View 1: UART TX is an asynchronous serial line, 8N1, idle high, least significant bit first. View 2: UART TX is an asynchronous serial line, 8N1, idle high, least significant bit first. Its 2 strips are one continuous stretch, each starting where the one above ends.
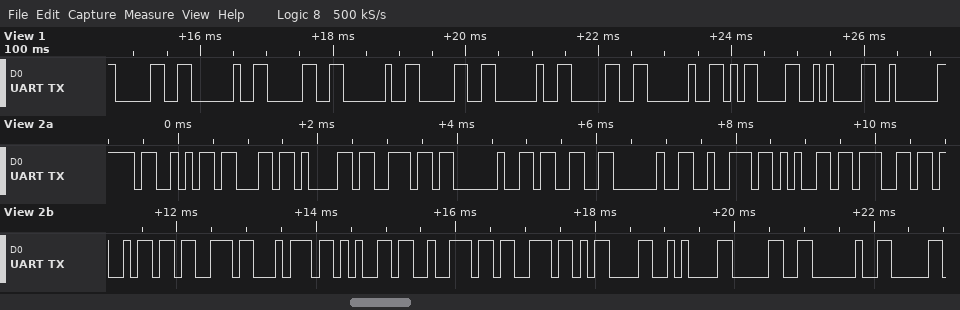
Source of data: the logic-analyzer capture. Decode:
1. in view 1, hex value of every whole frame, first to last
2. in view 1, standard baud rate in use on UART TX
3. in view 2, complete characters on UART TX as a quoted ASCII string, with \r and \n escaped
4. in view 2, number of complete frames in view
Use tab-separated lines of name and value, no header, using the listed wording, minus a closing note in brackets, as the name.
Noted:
in view 1, hex value of every whole frame, first to last	0x30 0x20 0x30 0x20 0x30 0x20 0x30 0x20 0x0D 0x0A 0x02
in view 1, standard baud rate in use on UART TX	9600 baud
in view 2, complete characters on UART TX as a quoted ASCII string, with \r and \n escaped	"Scan 3 registers\r\n0 "
in view 2, number of complete frames in view	20
